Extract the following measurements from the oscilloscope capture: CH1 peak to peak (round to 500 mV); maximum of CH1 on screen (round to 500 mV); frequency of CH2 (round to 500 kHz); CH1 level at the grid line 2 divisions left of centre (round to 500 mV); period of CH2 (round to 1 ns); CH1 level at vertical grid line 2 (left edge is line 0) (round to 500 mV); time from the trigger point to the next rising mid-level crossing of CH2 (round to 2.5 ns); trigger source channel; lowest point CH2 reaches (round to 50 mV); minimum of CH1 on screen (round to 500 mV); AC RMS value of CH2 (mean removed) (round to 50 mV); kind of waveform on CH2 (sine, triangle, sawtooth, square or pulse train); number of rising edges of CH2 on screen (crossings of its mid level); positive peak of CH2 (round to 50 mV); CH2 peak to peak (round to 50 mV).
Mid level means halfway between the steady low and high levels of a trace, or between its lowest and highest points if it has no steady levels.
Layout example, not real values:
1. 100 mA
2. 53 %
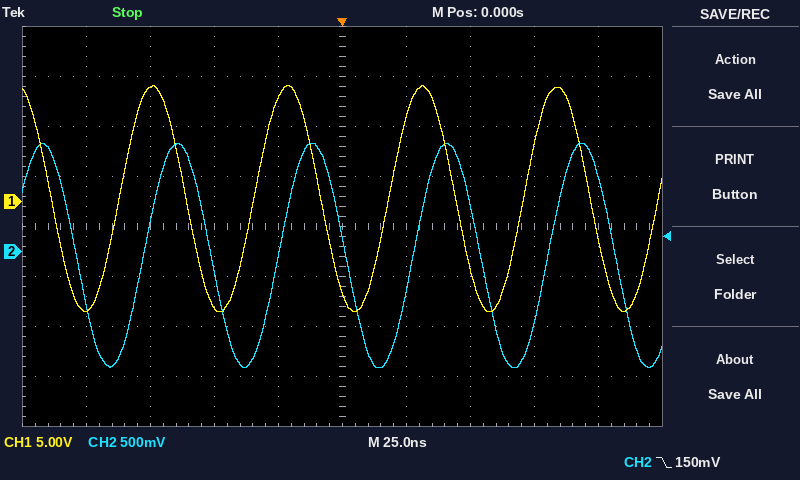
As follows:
1. 22.5 V
2. 11.5 V
3. 19.0 MHz
4. -10.5 V
5. 53 ns
6. 11.5 V
7. 27.5 ns
8. CH2
9. -1.15 V
10. -11.0 V
11. 800 mV
12. sine
13. 4
14. 1.10 V
15. 2.25 V
